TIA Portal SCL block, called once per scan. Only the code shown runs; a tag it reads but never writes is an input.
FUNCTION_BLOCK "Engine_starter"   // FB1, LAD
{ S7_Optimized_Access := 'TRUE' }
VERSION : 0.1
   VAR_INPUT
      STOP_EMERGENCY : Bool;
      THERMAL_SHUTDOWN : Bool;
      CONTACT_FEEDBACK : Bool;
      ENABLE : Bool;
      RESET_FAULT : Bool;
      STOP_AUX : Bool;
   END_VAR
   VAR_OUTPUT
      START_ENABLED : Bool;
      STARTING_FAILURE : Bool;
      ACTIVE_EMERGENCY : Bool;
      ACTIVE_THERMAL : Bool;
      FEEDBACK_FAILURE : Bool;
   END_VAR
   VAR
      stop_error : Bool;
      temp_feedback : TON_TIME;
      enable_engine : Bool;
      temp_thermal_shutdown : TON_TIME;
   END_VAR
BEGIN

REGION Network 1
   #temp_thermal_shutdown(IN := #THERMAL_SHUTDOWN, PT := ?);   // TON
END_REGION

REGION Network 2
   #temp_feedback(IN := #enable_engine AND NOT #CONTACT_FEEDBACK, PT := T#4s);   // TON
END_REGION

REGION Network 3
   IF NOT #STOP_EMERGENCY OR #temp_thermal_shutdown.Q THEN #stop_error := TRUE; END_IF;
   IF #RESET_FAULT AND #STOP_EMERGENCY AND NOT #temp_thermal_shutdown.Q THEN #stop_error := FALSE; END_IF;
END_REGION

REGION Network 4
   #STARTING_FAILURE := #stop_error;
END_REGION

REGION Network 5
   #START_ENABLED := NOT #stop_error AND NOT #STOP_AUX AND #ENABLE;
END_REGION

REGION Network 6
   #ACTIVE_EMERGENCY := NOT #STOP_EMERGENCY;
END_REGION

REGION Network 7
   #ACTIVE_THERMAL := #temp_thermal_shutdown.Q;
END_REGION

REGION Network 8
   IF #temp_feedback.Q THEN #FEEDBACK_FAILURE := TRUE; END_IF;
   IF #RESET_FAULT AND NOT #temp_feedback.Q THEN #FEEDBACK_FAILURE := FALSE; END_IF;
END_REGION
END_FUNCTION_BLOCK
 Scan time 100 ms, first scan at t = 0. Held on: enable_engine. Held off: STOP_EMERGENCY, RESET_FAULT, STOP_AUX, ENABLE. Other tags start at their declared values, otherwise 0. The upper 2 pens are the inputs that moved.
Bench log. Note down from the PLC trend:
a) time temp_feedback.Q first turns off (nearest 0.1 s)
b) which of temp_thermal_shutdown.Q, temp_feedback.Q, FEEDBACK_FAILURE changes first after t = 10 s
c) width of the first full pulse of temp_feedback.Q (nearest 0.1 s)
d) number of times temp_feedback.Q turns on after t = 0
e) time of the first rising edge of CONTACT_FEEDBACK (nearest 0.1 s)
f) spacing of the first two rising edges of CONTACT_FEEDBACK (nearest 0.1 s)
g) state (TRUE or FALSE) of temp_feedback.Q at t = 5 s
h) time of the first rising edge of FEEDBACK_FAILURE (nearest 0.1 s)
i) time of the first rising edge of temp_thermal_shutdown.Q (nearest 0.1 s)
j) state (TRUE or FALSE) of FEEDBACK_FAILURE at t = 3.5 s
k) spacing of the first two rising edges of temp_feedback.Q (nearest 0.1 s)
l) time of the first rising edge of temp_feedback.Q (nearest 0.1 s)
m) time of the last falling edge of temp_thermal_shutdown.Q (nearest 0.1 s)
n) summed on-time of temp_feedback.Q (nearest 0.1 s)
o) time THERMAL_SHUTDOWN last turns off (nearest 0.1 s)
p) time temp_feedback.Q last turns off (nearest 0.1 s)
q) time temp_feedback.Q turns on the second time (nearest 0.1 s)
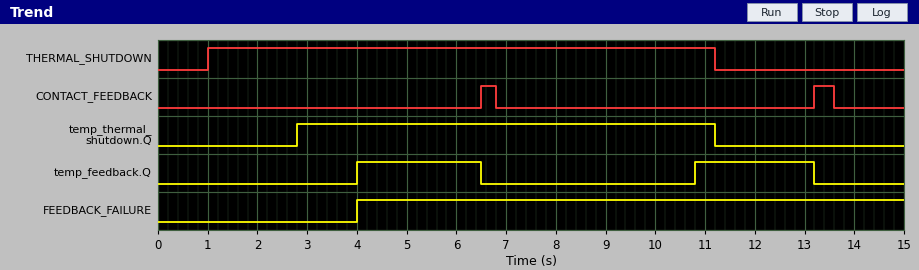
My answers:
6.5 s
temp_feedback.Q
2.5 s
2
6.5 s
6.7 s
TRUE
4.0 s
2.8 s
FALSE
6.8 s
4.0 s
11.2 s
4.9 s
11.2 s
13.2 s
10.8 s
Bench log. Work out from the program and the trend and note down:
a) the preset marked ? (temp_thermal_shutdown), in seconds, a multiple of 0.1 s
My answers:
1.8 s
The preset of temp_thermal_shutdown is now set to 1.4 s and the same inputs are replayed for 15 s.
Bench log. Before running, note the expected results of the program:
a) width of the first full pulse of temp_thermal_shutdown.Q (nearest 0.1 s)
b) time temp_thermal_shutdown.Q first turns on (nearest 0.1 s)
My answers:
8.8 s
2.4 s
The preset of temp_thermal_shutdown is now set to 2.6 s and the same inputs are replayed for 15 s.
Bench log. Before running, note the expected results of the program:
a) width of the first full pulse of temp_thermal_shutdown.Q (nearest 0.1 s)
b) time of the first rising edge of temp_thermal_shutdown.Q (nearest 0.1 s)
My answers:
7.6 s
3.6 s
